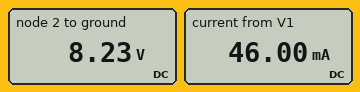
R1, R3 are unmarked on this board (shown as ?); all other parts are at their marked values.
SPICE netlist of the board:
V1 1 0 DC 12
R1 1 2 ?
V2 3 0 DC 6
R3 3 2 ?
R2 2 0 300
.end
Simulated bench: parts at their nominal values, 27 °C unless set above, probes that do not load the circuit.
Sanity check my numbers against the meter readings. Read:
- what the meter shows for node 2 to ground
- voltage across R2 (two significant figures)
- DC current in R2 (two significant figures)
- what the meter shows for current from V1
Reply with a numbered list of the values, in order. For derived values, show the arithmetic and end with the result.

1. 8.23 V
2. 8.23 V = 8.2 V
3. (8.23 V) / 300 Ω = 27 mA
4. 46.00 mA
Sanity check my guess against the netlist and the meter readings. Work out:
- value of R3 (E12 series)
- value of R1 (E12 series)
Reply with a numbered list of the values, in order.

1. 120 Ω
2. 82 Ω
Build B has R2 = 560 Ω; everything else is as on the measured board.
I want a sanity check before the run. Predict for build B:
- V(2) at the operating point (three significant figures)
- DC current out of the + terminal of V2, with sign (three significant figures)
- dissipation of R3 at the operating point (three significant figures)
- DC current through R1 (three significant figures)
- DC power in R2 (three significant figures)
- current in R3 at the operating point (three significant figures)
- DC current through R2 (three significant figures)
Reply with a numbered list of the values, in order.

1. 8.80 V
2. -23.3 mA
3. 65.3 mW
4. 39.0 mA
5. 138 mW
6. 23.3 mA
7. 15.7 mA
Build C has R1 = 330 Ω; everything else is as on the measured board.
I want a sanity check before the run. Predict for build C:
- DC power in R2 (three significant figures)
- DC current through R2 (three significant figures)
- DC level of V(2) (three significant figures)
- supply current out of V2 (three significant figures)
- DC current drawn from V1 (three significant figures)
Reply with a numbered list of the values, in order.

1. 115 mW
2. 19.6 mA
3. 5.88 V
4. 1.03 mA
5. 18.6 mA
